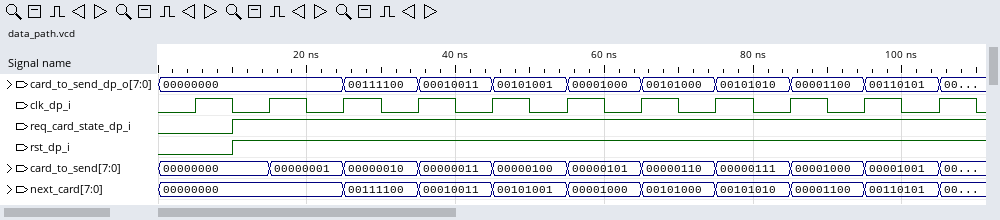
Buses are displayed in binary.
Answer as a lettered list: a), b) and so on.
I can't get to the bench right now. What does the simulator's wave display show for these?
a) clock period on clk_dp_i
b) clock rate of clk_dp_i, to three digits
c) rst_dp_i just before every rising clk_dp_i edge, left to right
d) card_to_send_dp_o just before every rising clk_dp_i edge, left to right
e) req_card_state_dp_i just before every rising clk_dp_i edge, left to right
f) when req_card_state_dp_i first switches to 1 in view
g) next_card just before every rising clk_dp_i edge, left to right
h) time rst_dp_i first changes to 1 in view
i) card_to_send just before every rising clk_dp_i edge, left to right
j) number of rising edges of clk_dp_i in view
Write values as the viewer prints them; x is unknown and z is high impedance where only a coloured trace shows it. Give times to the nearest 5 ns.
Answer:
a) 10 ns
b) 100 MHz
c) 0 1 1 1 1 1 1 1 1 1 1
d) 00000000, 00000000, 00000000, 00111100, 00010011, 00101001, 00001000, 00101000, 00101010, 00001100, 00110101
e) 0 1 1 1 1 1 1 1 1 1 1
f) 10 ns
g) 00000000, 00000000, 00000000, 00111100, 00010011, 00101001, 00001000, 00101000, 00101010, 00001100, 00110101
h) 10 ns
i) 00000000, 00000000, 00000001, 00000010, 00000011, 00000100, 00000101, 00000110, 00000111, 00001000, 00001001
j) 11
